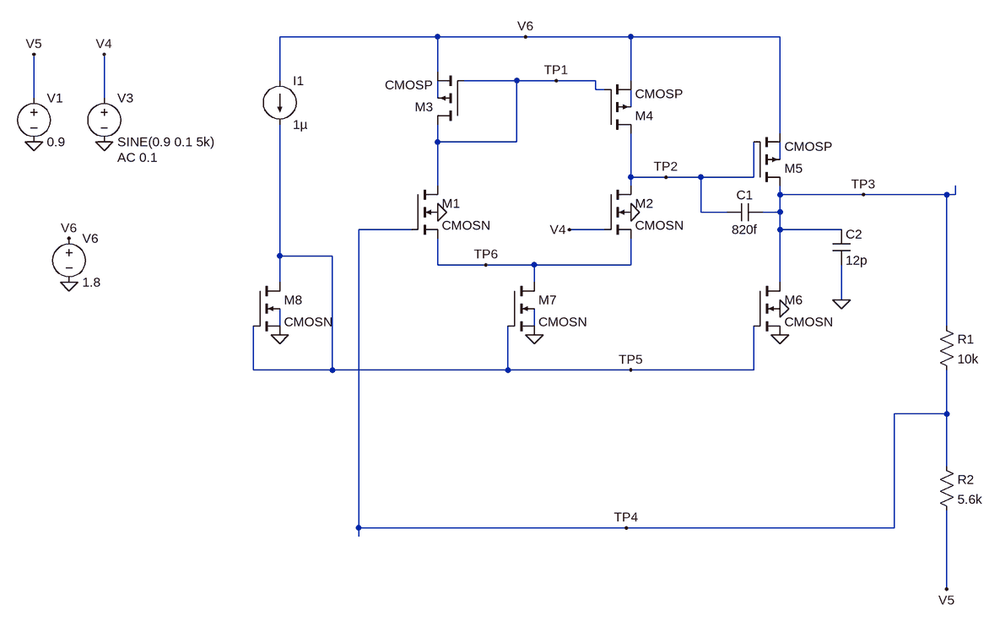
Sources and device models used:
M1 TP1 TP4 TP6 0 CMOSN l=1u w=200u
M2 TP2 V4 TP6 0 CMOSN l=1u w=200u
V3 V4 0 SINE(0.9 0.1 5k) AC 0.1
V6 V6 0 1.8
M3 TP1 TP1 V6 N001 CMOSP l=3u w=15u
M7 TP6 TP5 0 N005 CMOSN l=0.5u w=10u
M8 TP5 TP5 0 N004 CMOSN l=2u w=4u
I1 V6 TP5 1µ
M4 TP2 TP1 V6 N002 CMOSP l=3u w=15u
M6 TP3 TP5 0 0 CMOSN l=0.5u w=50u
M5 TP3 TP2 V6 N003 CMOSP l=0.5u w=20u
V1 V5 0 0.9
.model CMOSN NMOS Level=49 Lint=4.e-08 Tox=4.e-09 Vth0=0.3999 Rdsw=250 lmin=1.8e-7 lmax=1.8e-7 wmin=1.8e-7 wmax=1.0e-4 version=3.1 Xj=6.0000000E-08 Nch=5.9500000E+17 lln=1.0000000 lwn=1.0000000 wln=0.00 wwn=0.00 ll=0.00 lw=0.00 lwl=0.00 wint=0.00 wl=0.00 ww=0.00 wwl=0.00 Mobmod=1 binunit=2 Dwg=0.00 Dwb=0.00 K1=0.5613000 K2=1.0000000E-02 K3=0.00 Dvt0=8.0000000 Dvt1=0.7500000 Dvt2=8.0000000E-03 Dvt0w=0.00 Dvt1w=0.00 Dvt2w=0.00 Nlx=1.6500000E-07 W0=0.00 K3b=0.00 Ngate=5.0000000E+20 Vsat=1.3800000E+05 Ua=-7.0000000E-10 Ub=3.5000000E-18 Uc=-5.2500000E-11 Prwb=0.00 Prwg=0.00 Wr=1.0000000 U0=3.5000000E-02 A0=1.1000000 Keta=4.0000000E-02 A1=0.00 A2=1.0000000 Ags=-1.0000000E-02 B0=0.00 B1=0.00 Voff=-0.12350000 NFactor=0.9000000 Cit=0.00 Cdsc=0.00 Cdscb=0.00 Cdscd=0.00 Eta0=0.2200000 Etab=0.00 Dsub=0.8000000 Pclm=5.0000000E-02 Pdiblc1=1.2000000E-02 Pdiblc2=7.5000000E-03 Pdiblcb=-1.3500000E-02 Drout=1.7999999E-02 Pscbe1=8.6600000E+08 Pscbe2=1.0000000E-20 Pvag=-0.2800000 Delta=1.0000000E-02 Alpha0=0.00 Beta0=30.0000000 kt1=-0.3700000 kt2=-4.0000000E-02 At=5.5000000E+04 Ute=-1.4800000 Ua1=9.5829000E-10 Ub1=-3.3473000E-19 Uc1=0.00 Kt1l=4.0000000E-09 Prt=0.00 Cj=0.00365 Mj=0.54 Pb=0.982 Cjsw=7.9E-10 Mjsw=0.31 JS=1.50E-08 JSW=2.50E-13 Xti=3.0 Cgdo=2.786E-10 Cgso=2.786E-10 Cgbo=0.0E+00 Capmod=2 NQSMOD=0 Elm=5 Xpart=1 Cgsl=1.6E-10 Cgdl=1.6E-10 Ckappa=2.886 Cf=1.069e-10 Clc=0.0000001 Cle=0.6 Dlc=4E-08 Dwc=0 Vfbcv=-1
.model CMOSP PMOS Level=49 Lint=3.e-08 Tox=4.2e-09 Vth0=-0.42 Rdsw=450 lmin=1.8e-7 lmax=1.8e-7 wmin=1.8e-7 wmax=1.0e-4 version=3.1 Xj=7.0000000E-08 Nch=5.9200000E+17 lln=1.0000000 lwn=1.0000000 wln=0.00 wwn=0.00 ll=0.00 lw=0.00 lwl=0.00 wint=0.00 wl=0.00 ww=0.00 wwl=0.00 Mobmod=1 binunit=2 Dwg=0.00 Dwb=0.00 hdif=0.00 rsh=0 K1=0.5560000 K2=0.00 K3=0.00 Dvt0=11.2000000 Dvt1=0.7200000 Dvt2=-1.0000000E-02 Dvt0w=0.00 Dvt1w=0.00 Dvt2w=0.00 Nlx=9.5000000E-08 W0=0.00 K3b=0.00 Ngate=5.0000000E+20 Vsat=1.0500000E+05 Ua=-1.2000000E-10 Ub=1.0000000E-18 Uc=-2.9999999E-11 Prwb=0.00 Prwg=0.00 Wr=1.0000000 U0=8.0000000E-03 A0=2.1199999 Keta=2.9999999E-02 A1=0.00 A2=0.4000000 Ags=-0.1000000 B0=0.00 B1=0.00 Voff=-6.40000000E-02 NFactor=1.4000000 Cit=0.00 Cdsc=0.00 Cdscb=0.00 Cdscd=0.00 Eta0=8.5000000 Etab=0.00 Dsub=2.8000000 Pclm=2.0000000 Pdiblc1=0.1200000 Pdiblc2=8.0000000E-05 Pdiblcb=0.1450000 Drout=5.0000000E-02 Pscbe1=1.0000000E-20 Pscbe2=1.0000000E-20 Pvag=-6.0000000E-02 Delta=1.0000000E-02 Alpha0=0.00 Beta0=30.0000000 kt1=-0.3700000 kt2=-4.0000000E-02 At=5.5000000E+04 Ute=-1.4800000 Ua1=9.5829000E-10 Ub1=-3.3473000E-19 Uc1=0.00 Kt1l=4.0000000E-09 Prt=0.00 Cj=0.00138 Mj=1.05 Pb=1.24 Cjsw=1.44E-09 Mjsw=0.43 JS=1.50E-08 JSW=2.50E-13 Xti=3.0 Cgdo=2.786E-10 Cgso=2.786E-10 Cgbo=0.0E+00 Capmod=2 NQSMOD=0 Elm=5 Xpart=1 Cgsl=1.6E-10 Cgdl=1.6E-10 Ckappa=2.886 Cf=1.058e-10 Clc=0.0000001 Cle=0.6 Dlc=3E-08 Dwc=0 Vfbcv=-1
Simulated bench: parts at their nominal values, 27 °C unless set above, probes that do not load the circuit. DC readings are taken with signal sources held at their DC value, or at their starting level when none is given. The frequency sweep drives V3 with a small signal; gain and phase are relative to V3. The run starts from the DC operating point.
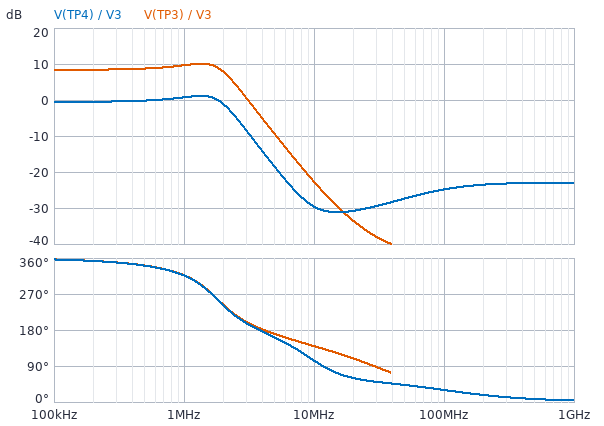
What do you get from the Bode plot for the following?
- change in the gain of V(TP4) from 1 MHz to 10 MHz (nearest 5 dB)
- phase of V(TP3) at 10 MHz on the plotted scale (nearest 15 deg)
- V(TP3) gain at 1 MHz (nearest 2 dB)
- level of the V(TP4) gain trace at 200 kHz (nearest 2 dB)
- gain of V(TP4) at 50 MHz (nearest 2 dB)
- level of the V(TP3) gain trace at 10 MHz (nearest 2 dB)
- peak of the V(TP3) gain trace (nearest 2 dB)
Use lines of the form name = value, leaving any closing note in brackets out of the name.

change in the gain of V(TP4) from 1 MHz to 10 MHz = -30 dB
phase of V(TP3) at 10 MHz on the plotted scale = 135 deg
V(TP3) gain at 1 MHz = 10 dB
level of the V(TP4) gain trace at 200 kHz = 0 dB
gain of V(TP4) at 50 MHz = -28 dB
level of the V(TP3) gain trace at 10 MHz = -22 dB
peak of the V(TP3) gain trace = 10 dB
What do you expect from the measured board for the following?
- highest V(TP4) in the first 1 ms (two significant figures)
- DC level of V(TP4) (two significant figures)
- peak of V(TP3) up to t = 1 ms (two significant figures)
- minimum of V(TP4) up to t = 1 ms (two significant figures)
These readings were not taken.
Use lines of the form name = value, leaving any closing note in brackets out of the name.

highest V(TP4) in the first 1 ms = 1.0 V
DC level of V(TP4) = 900 mV
peak of V(TP3) up to t = 1 ms = 1.2 V
minimum of V(TP4) up to t = 1 ms = 870 mV
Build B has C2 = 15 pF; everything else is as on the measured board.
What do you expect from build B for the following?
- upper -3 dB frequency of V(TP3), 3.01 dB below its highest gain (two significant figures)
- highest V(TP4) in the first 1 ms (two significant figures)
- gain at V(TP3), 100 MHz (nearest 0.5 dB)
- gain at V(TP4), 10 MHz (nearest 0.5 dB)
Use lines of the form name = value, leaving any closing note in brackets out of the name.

upper -3 dB frequency of V(TP3), 3.01 dB below its highest gain = 1.9 MHz
highest V(TP4) in the first 1 ms = 1.0 V
gain at V(TP3), 100 MHz = -45.5 dB
gain at V(TP4), 10 MHz = -30.5 dB
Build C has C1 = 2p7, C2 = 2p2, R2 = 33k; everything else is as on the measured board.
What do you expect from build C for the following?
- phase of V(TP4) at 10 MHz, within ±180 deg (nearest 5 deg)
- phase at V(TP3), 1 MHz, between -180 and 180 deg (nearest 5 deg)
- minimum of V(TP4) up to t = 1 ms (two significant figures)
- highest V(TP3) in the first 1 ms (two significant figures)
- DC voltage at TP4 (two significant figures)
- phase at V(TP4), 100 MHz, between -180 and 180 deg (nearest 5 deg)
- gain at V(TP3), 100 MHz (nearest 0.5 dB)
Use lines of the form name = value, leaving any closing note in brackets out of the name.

phase of V(TP4) at 10 MHz, within ±180 deg = 90 deg
phase at V(TP3), 1 MHz, between -180 and 180 deg = -40 deg
minimum of V(TP4) up to t = 1 ms = 800 mV
highest V(TP3) in the first 1 ms = 1.0 V
DC voltage at TP4 = 900 mV
phase at V(TP4), 100 MHz, between -180 and 180 deg = 5 deg
gain at V(TP3), 100 MHz = -28.5 dB
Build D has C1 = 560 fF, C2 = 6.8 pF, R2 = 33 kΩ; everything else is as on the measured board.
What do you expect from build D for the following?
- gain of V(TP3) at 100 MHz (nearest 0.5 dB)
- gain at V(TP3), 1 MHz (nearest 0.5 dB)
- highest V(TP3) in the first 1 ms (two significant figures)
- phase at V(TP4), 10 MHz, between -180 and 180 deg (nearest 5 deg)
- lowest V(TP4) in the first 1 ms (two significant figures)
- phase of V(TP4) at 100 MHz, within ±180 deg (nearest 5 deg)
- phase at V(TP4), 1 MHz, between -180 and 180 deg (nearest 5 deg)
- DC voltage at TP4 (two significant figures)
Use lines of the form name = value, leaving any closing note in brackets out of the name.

gain of V(TP3) at 100 MHz = -40.0 dB
gain at V(TP3), 1 MHz = 3.0 dB
highest V(TP3) in the first 1 ms = 1.0 V
phase at V(TP4), 10 MHz, between -180 and 180 deg = 110 deg
lowest V(TP4) in the first 1 ms = 800 mV
phase of V(TP4) at 100 MHz, within ±180 deg = 10 deg
phase at V(TP4), 1 MHz, between -180 and 180 deg = -10 deg
DC voltage at TP4 = 900 mV
